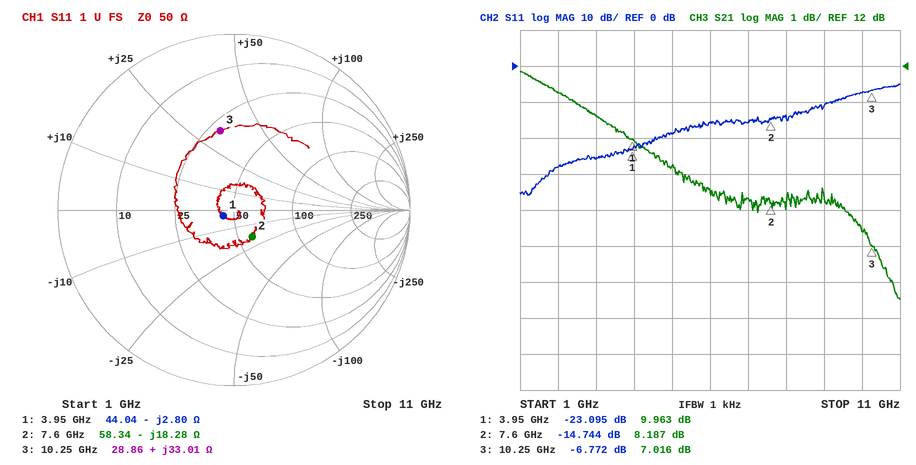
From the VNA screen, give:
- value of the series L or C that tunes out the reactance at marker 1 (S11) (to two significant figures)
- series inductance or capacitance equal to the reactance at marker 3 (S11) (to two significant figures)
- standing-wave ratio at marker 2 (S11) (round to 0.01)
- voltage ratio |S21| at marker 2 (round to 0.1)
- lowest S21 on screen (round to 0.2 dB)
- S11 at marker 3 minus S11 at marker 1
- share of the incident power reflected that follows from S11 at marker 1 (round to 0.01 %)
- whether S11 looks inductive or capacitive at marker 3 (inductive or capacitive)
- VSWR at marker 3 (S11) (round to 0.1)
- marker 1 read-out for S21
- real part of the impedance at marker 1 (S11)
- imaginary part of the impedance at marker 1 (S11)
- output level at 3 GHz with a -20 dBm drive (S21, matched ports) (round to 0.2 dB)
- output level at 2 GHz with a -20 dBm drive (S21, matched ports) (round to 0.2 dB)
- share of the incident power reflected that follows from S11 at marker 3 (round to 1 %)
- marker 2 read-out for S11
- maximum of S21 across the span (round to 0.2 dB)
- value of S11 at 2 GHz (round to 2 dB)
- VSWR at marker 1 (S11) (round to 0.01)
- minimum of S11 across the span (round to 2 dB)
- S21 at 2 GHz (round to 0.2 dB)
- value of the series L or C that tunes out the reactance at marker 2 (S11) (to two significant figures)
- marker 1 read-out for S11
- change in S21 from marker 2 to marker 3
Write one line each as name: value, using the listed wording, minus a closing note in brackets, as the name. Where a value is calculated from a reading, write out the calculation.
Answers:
value of the series L or C that tunes out the reactance at marker 1 (S11): L = 2.8 Ω/(2π × 3.95 GHz) ≈ 113 pH, so 110 pH to two significant figures
series inductance or capacitance equal to the reactance at marker 3 (S11): L = 33.01 Ω/(2π × 10.25 GHz) ≈ 513 pH, so 510 pH to two significant figures
standing-wave ratio at marker 2 (S11): 1.45
voltage ratio |S21| at marker 2: 10^(8.187/20) ≈ 2.6
lowest S21 on screen: 5.6 dB
S11 at marker 3 minus S11 at marker 1: -6.772 − (-23.095) = 16.323 dB
share of the incident power reflected that follows from S11 at marker 1: 10^(-23.095/10) ≈ 0.49 %
whether S11 looks inductive or capacitive at marker 3: inductive
VSWR at marker 3 (S11): 2.7
marker 1 read-out for S21: 9.963 dB
real part of the impedance at marker 1: 44.04 Ω
imaginary part of the impedance at marker 1: -2.80 Ω
output level at 3 GHz with a -20 dBm drive (S21, matched ports): -20 dBm + (10.6 dB) = -9.4 dBm
output level at 2 GHz with a -20 dBm drive (S21, matched ports): -20 dBm + (11.2 dB) = -8.8 dBm
share of the incident power reflected that follows from S11 at marker 3: 10^(-6.772/10) ≈ 21 %
marker 2 read-out for S11: -14.744 dB
maximum of S21 across the span: 11.8 dB
value of S11 at 2 GHz: -28 dB
VSWR at marker 1 (S11): 1.15
minimum of S11 across the span: -36 dB
S21 at 2 GHz: 11.2 dB
value of the series L or C that tunes out the reactance at marker 2 (S11): L = 18.28 Ω/(2π × 7.6 GHz) ≈ 383 pH, so 380 pH to two significant figures
marker 1 read-out for S11: -23.095 dB
change in S21 from marker 2 to marker 3: 7.016 − (8.187) = -1.171 dB
